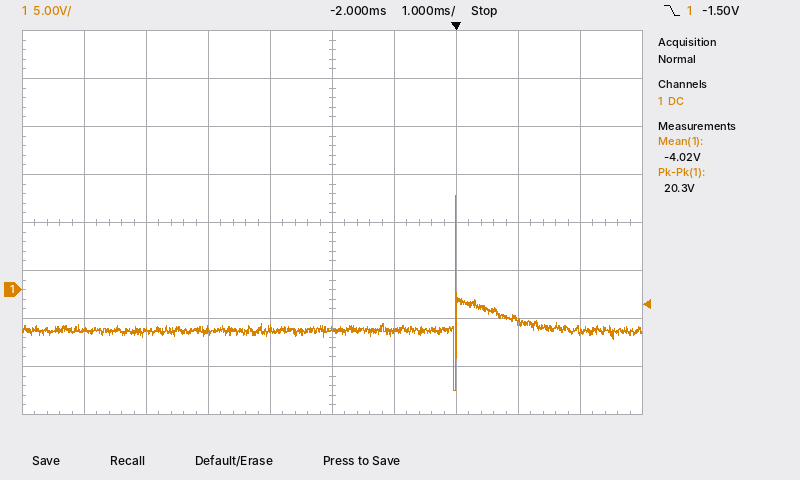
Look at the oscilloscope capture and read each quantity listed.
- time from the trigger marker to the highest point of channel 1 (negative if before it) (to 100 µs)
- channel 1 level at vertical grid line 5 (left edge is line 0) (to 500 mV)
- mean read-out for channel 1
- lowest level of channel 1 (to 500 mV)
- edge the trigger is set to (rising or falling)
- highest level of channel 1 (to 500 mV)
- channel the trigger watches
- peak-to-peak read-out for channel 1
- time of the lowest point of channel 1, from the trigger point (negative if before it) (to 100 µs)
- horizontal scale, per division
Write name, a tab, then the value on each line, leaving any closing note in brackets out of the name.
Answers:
time from the trigger marker to the highest point of channel 1 (negative if before it)	0.0 ms
channel 1 level at vertical grid line 5 (left edge is line 0)	-4.0 V
mean read-out for channel 1	-4.02 V
lowest level of channel 1	-10.5 V
edge the trigger is set to	falling
highest level of channel 1	10.0 V
channel the trigger watches	channel 1
peak-to-peak read-out for channel 1	20.3 V
time of the lowest point of channel 1, from the trigger point (negative if before it)	0.0 ms
horizontal scale, per division	1 ms
